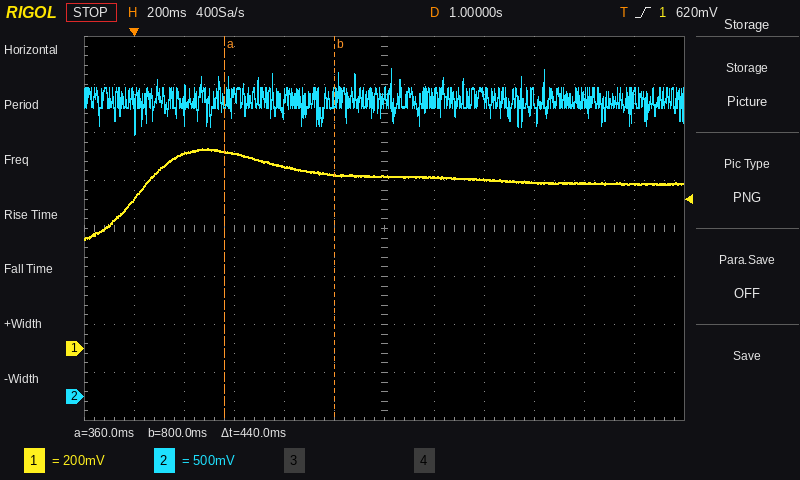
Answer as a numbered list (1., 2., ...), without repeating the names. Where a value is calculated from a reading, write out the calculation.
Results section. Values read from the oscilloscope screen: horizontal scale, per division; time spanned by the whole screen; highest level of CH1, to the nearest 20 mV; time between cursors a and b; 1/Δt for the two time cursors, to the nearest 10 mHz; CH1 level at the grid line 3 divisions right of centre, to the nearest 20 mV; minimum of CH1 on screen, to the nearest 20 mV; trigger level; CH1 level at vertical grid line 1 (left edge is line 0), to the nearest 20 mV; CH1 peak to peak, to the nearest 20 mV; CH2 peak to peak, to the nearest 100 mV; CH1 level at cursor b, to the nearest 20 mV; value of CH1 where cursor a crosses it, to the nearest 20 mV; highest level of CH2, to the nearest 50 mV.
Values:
1. 200 ms
2. 2.4 s
3. 840 mV
4. 440 ms
5. 1 / 440 ms ≈ 2.27 Hz
6. 700 mV
7. 460 mV
8. 620 mV
9. 620 mV
10. 840 mV − (460 mV) = 380 mV
11. 700 mV
12. 720 mV
13. 820 mV
14. 3.40 V
